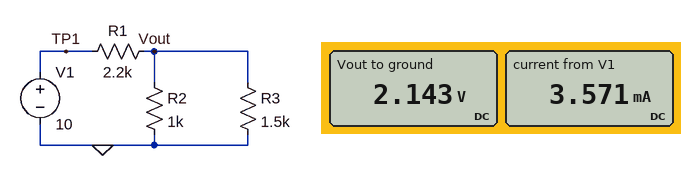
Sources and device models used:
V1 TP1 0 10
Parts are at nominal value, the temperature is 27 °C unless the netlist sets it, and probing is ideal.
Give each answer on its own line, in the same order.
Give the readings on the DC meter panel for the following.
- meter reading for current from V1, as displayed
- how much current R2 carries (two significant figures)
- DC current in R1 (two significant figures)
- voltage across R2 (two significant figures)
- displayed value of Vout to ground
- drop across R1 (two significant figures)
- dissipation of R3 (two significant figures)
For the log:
3.571 mA
2.1 mA
3.6 mA
2.1 V
2.143 V
7.9 V
3.1 mW
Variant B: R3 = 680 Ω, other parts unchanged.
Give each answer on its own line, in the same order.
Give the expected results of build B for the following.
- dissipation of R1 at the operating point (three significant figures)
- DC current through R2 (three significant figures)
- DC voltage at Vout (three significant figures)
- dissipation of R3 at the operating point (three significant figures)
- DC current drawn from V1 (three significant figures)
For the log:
32.4 mW
1.55 mA
1.55 V
3.55 mW
3.84 mA
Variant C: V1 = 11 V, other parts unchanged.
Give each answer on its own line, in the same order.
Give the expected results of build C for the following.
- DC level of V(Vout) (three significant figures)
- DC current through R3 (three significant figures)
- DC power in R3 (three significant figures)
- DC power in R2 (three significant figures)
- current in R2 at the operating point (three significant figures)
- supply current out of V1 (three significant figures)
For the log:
2.36 V
1.57 mA
3.70 mW
5.56 mW
2.36 mA
3.93 mA
